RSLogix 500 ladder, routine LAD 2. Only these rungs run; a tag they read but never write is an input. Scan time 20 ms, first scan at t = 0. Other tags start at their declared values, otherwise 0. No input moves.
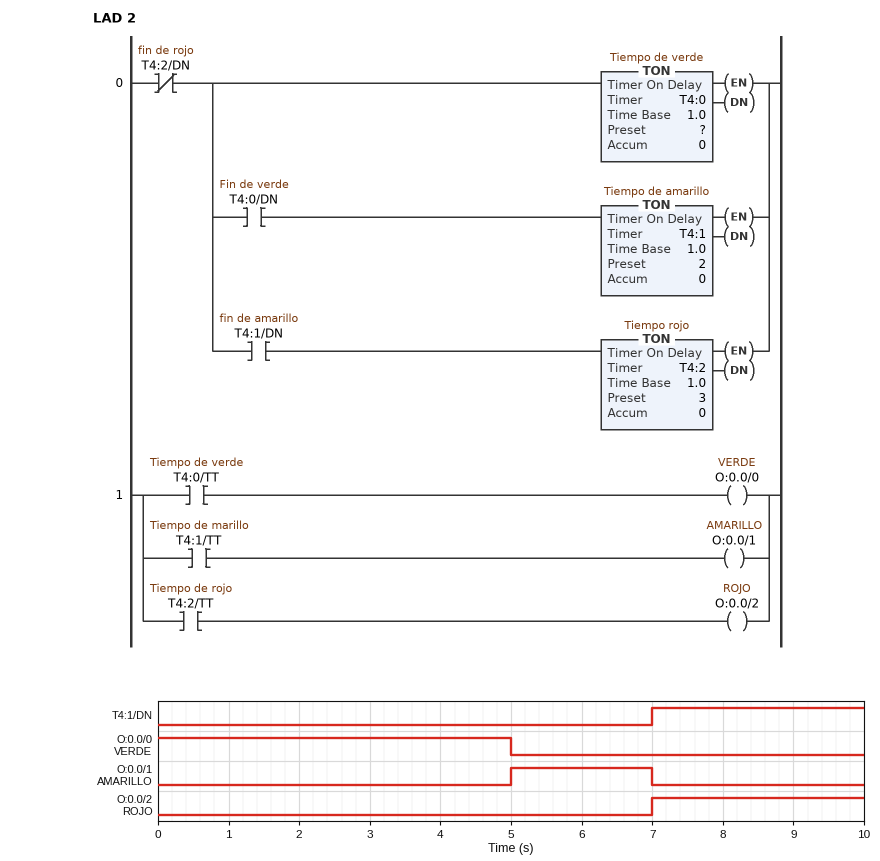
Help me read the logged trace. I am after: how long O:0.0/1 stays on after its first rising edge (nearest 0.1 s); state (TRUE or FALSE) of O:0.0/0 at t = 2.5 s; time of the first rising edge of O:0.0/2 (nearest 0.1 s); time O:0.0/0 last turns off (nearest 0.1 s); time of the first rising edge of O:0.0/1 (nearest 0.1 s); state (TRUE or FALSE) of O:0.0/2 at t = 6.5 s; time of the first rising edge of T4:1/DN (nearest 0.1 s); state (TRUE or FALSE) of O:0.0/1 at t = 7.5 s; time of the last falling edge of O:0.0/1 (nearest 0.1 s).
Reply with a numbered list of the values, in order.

1. 2.0 s
2. TRUE
3. 7.0 s
4. 5.0 s
5. 5.0 s
6. FALSE
7. 7.0 s
8. FALSE
9. 7.0 s
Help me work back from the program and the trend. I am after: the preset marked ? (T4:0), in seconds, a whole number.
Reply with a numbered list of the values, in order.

1. 5 s
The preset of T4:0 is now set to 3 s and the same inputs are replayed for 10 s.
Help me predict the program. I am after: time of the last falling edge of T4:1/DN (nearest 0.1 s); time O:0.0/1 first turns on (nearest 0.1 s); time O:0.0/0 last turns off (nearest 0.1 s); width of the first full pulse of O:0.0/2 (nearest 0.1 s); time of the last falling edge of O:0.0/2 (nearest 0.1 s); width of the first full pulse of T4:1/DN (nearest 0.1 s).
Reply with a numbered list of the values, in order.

1. 8.0 s
2. 3.0 s
3. 3.0 s
4. 3.0 s
5. 8.0 s
6. 3.0 s
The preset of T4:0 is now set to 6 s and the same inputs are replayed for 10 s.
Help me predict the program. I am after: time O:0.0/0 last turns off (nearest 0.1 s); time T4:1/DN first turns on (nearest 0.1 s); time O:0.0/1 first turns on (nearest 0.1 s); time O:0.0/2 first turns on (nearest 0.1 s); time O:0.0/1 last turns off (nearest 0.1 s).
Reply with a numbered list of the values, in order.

1. 6.0 s
2. 8.0 s
3. 6.0 s
4. 8.0 s
5. 8.0 s
